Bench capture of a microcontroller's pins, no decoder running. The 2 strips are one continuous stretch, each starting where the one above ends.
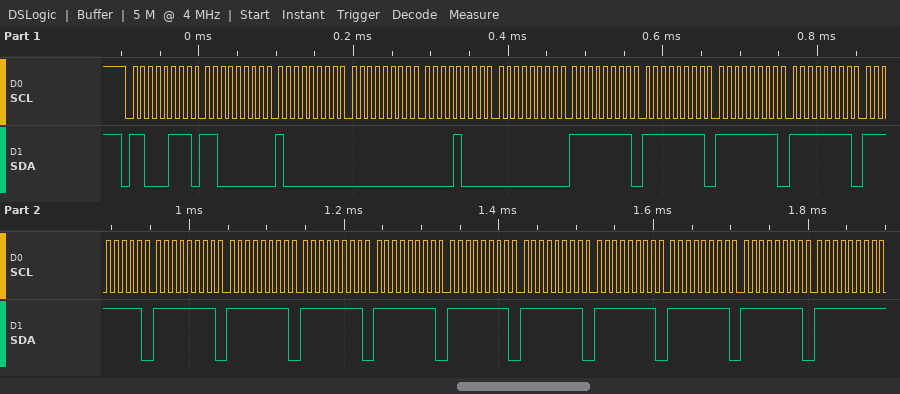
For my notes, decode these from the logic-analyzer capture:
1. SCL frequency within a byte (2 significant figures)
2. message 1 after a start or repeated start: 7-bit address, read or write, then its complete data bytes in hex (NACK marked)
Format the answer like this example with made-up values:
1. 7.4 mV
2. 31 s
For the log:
1. 100 kHz
2. 0x63 read: C0 80 00 08 00 FF FF FF FF FF FF FF FF FF FF FF FF FF FF FF NACK
